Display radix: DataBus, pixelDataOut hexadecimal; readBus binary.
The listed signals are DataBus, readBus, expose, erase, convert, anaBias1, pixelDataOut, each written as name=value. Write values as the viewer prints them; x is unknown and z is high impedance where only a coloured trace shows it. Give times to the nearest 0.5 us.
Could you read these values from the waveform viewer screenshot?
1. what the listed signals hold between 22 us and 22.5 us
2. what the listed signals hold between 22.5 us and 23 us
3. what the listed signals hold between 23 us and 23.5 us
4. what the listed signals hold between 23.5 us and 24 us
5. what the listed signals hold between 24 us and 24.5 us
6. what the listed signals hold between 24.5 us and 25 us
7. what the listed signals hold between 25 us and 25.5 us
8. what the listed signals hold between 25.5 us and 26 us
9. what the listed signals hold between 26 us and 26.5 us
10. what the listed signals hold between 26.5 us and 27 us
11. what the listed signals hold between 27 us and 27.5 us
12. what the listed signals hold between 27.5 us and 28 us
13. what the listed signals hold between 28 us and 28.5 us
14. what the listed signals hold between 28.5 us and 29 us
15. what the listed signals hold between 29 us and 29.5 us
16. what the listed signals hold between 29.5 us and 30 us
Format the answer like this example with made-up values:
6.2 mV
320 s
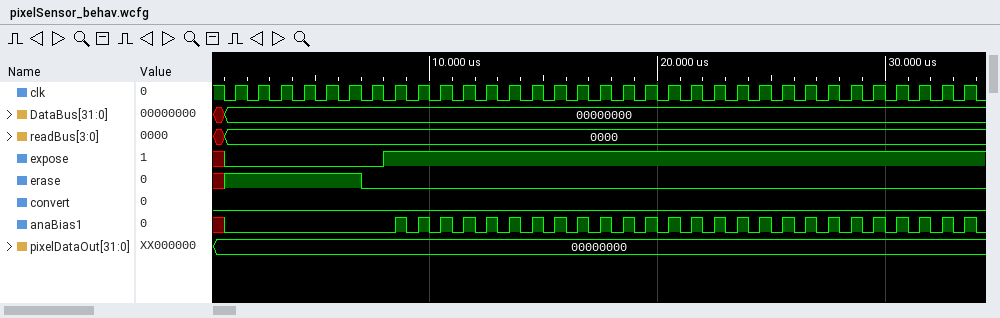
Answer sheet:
DataBus=00000000, readBus=0000, expose=1, erase=0, convert=0, anaBias1=0, pixelDataOut=00000000
DataBus=00000000, readBus=0000, expose=1, erase=0, convert=0, anaBias1=1, pixelDataOut=00000000
DataBus=00000000, readBus=0000, expose=1, erase=0, convert=0, anaBias1=0, pixelDataOut=00000000
DataBus=00000000, readBus=0000, expose=1, erase=0, convert=0, anaBias1=1, pixelDataOut=00000000
DataBus=00000000, readBus=0000, expose=1, erase=0, convert=0, anaBias1=0, pixelDataOut=00000000
DataBus=00000000, readBus=0000, expose=1, erase=0, convert=0, anaBias1=1, pixelDataOut=00000000
DataBus=00000000, readBus=0000, expose=1, erase=0, convert=0, anaBias1=0, pixelDataOut=00000000
DataBus=00000000, readBus=0000, expose=1, erase=0, convert=0, anaBias1=1, pixelDataOut=00000000
DataBus=00000000, readBus=0000, expose=1, erase=0, convert=0, anaBias1=0, pixelDataOut=00000000
DataBus=00000000, readBus=0000, expose=1, erase=0, convert=0, anaBias1=1, pixelDataOut=00000000
DataBus=00000000, readBus=0000, expose=1, erase=0, convert=0, anaBias1=0, pixelDataOut=00000000
DataBus=00000000, readBus=0000, expose=1, erase=0, convert=0, anaBias1=1, pixelDataOut=00000000
DataBus=00000000, readBus=0000, expose=1, erase=0, convert=0, anaBias1=0, pixelDataOut=00000000
DataBus=00000000, readBus=0000, expose=1, erase=0, convert=0, anaBias1=1, pixelDataOut=00000000
DataBus=00000000, readBus=0000, expose=1, erase=0, convert=0, anaBias1=0, pixelDataOut=00000000
DataBus=00000000, readBus=0000, expose=1, erase=0, convert=0, anaBias1=1, pixelDataOut=00000000
